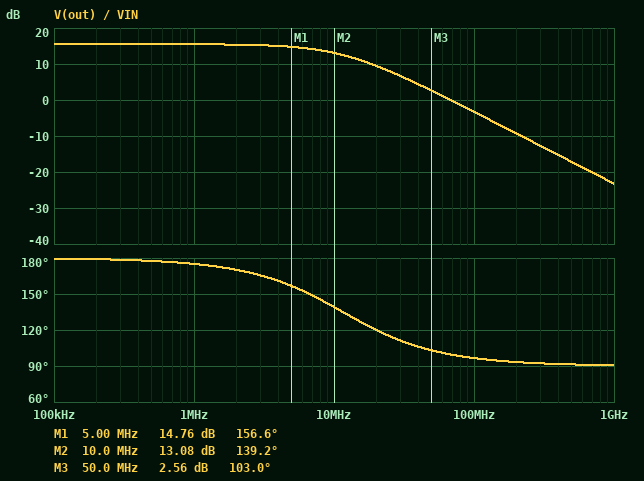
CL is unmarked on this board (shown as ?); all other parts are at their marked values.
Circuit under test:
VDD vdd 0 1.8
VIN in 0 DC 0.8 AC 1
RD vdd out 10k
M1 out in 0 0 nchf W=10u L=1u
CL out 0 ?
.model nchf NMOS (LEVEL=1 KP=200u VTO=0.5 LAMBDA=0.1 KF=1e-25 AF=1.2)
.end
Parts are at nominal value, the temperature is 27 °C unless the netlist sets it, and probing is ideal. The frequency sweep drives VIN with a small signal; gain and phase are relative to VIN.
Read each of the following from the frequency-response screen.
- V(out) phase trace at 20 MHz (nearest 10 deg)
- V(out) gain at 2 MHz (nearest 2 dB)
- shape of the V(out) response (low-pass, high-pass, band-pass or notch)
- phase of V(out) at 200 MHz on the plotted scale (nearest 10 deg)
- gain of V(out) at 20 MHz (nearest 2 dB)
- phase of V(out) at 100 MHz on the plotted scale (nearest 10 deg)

120 deg
16 dB
low-pass
90 deg
10 dB
100 deg
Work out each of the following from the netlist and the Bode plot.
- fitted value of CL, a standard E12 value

1.5 pF
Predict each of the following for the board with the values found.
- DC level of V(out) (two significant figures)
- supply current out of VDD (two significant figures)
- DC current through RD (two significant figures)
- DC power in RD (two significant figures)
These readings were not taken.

830 mV
97 µA
97 µA
95 µW
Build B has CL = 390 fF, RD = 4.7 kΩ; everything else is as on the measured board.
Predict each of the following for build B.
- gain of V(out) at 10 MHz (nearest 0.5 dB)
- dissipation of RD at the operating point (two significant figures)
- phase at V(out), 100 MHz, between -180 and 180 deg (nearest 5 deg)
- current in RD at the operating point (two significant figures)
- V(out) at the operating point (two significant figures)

9.5 dB
49 µW
130 deg
100 µA
1.3 V
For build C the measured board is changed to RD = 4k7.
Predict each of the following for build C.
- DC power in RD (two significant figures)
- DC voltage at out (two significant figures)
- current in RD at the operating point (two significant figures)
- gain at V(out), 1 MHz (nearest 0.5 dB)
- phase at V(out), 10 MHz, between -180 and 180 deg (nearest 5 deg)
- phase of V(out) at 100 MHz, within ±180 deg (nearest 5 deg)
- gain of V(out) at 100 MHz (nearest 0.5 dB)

49 µW
1.3 V
100 µA
9.5 dB
155 deg
105 deg
-3.0 dB
